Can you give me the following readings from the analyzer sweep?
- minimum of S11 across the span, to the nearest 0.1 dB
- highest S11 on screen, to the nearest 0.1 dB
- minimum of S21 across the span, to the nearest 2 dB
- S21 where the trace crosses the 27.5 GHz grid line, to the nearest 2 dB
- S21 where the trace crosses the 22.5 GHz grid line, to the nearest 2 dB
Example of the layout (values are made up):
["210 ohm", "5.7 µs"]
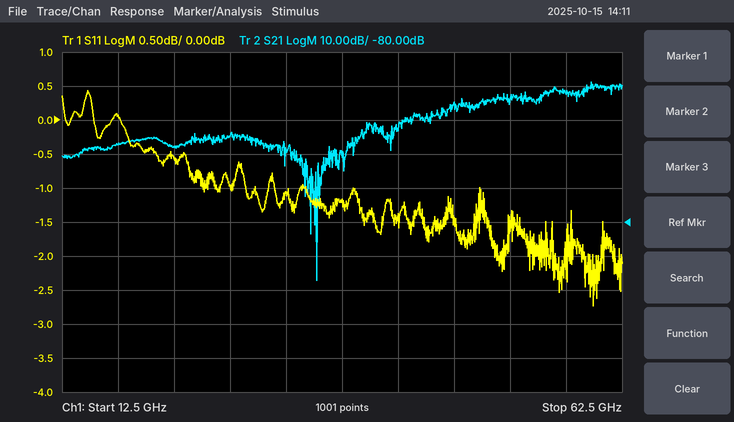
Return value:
["-2.7 dB", "0.4 dB", "-98 dB", "-54 dB", "-58 dB"]
